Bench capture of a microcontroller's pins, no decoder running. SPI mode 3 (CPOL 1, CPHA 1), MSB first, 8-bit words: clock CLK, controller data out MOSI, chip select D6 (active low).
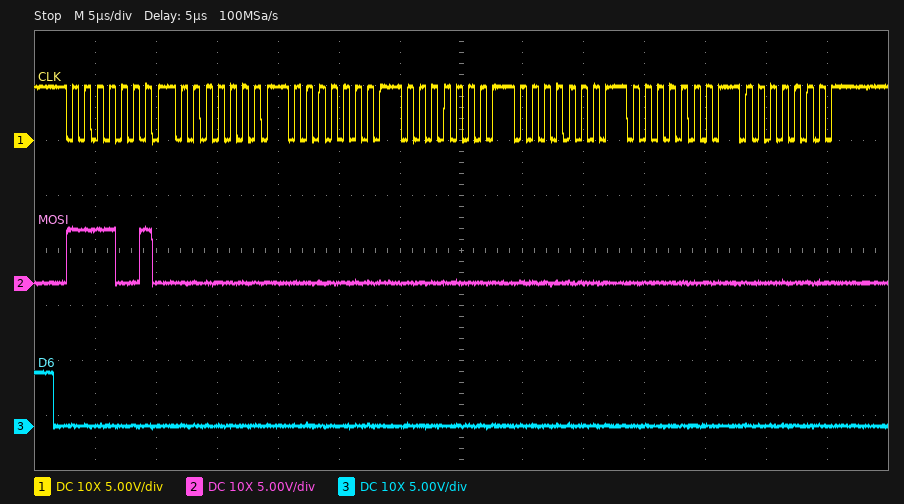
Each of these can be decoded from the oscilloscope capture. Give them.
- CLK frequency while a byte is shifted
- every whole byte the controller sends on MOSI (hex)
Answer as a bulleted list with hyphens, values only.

- 1 MHz
- 0xF2 0x00 0x00 0x00 0x00 0x00 0x00
